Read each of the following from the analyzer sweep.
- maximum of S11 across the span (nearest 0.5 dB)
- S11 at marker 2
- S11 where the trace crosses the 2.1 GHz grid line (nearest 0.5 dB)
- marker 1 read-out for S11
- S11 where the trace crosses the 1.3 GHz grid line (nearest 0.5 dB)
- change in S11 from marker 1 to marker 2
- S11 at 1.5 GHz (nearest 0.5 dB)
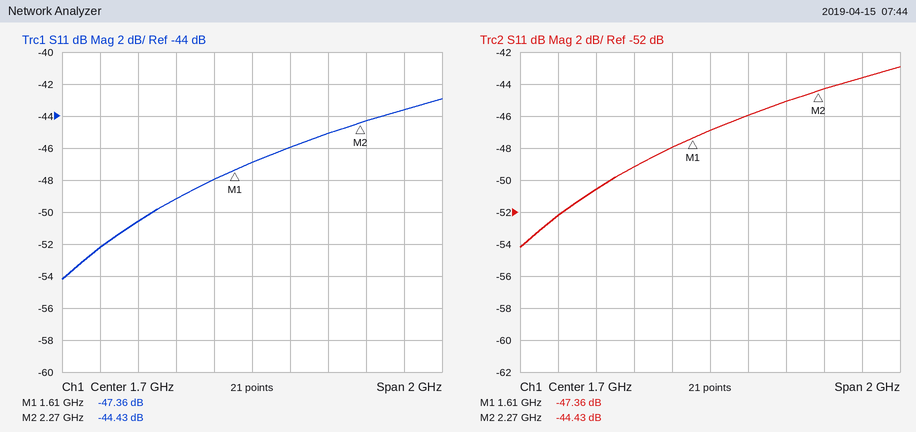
-43.0 dB
-44.43 dB
-45.0 dB
-47.36 dB
-49.0 dB
2.93 dB
-48.0 dB
